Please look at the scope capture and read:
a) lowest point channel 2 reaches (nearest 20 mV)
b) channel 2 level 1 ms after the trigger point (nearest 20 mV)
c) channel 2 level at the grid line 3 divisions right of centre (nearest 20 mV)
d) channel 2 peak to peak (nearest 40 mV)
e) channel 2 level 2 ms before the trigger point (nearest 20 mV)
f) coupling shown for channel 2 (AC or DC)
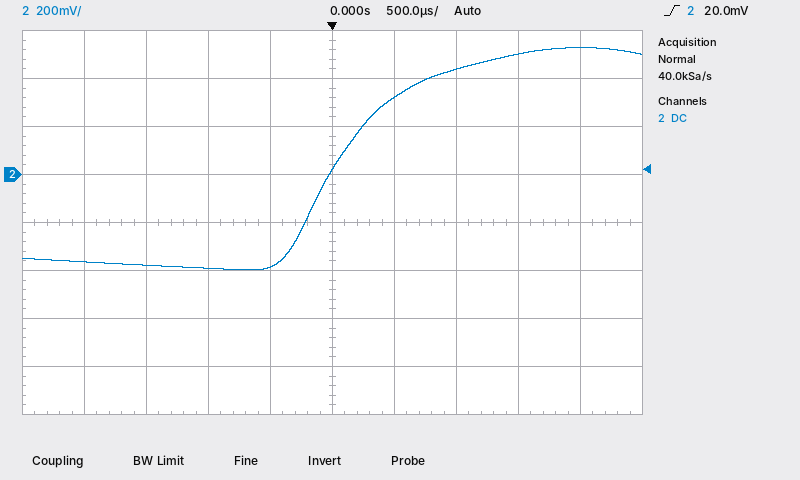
-400 mV
440 mV
500 mV
920 mV
-360 mV
DC
